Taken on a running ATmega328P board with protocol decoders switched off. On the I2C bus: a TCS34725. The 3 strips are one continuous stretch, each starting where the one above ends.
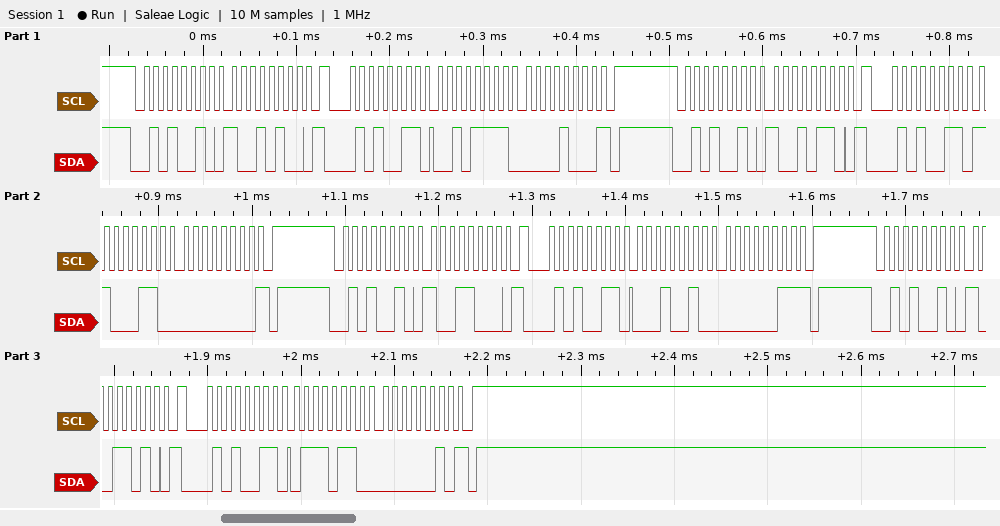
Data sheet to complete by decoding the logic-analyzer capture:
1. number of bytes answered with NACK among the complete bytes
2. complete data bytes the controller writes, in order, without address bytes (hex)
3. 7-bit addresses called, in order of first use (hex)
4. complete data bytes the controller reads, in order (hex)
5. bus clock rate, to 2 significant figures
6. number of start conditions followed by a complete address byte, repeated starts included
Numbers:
4
94 96 98 9A
0x29
2F 08 C6 00 12 03 76 02
100 kHz
8
